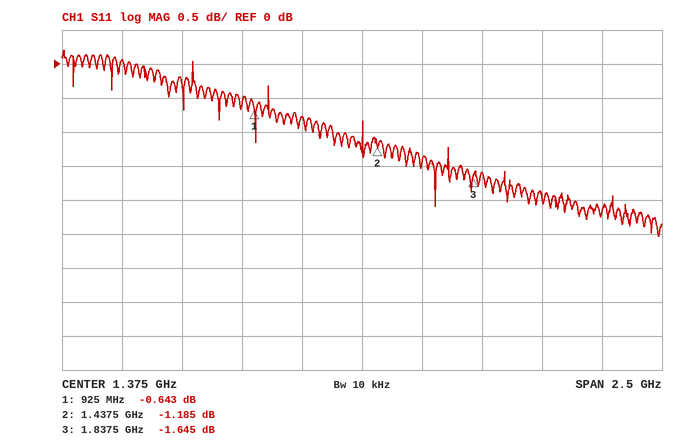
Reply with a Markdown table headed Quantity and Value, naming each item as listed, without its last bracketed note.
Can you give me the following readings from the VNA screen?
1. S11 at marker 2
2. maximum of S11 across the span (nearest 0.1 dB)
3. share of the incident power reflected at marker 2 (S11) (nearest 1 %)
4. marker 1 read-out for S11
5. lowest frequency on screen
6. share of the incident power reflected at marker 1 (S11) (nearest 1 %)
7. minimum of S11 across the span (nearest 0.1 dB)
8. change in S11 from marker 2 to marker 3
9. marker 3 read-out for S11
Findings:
| Quantity | Value |
|---|---|
| S11 at marker 2 | -1.185 dB |
| maximum of S11 across the span | 0.2 dB |
| share of the incident power reflected at marker 2 (S11) | 76 % |
| marker 1 read-out for S11 | -0.643 dB |
| lowest frequency on screen | 125 MHz |
| share of the incident power reflected at marker 1 (S11) | 86 % |
| minimum of S11 across the span | -2.5 dB |
| change in S11 from marker 2 to marker 3 | -0.460 dB |
| marker 3 read-out for S11 | -1.645 dB |
